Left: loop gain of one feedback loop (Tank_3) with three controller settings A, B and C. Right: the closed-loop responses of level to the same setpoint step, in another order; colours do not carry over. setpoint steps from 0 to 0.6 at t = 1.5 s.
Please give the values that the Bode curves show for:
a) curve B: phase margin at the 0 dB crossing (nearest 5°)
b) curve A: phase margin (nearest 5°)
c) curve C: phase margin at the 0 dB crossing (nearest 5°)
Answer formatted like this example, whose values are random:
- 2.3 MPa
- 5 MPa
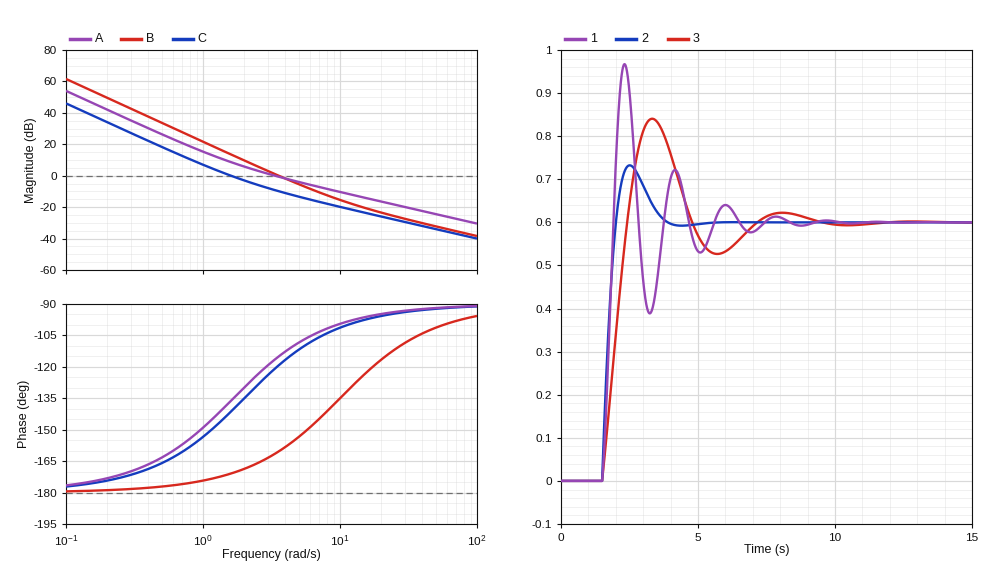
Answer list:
- 20°
- 65°
- 40°
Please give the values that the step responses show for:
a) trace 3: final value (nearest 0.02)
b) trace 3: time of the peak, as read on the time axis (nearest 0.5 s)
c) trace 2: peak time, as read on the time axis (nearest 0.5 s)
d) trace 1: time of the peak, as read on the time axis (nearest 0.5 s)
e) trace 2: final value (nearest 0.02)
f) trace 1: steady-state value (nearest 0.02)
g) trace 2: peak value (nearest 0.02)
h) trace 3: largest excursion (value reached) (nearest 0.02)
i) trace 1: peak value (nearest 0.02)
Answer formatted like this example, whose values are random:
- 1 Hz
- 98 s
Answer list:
- 0.60
- 3.5 s
- 2.5 s
- 2.5 s
- 0.60
- 0.60
- 0.74
- 0.84
- 0.96
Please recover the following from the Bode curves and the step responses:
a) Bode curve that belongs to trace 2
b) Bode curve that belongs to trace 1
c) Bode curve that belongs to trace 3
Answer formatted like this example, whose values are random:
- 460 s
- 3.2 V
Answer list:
- A
- B
- C
